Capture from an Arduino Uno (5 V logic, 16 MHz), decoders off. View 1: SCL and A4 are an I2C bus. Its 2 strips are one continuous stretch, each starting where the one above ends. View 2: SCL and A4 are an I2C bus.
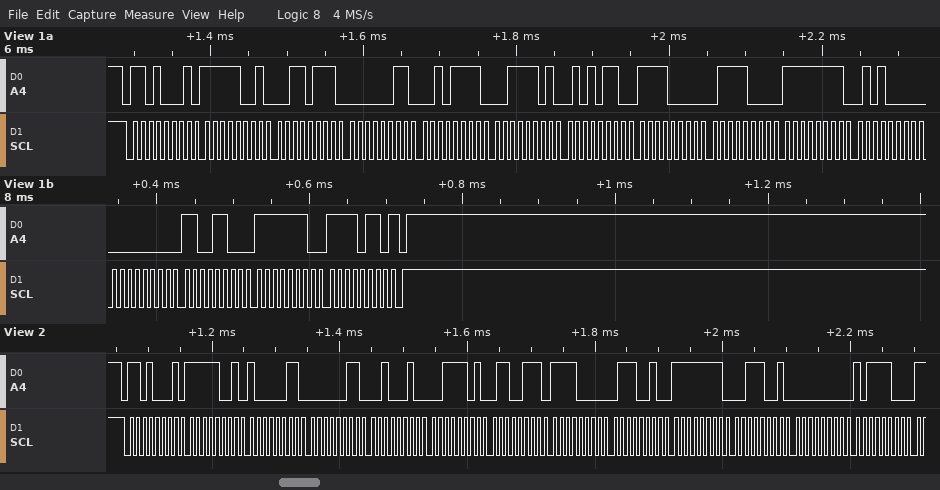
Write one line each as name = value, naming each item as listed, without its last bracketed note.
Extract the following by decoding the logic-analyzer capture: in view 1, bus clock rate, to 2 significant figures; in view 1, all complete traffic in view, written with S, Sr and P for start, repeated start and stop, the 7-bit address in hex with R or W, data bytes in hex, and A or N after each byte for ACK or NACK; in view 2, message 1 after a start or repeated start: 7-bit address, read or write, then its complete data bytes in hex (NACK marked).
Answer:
in view 1, bus clock rate, to 2 significant figures = 100 kHz
in view 1, all complete traffic in view, written with S, Sr and P for start, repeated start and stop, the 7-bit address in hex with R or W, data bytes in hex, and A or N after each byte for ACK or NACK = S 68R A F9 A 37 A 03 A 2F A 3D A 56 A F0 A 78 A FF A 50 A 00 A CC A FE A F6 N P
in view 2, message 1 after a start or repeated start: 7-bit address, read or write, then its complete data bytes in hex = 0x68 read: F9 83 03 22 3D 67 F0 72 FF 39 00 BC
